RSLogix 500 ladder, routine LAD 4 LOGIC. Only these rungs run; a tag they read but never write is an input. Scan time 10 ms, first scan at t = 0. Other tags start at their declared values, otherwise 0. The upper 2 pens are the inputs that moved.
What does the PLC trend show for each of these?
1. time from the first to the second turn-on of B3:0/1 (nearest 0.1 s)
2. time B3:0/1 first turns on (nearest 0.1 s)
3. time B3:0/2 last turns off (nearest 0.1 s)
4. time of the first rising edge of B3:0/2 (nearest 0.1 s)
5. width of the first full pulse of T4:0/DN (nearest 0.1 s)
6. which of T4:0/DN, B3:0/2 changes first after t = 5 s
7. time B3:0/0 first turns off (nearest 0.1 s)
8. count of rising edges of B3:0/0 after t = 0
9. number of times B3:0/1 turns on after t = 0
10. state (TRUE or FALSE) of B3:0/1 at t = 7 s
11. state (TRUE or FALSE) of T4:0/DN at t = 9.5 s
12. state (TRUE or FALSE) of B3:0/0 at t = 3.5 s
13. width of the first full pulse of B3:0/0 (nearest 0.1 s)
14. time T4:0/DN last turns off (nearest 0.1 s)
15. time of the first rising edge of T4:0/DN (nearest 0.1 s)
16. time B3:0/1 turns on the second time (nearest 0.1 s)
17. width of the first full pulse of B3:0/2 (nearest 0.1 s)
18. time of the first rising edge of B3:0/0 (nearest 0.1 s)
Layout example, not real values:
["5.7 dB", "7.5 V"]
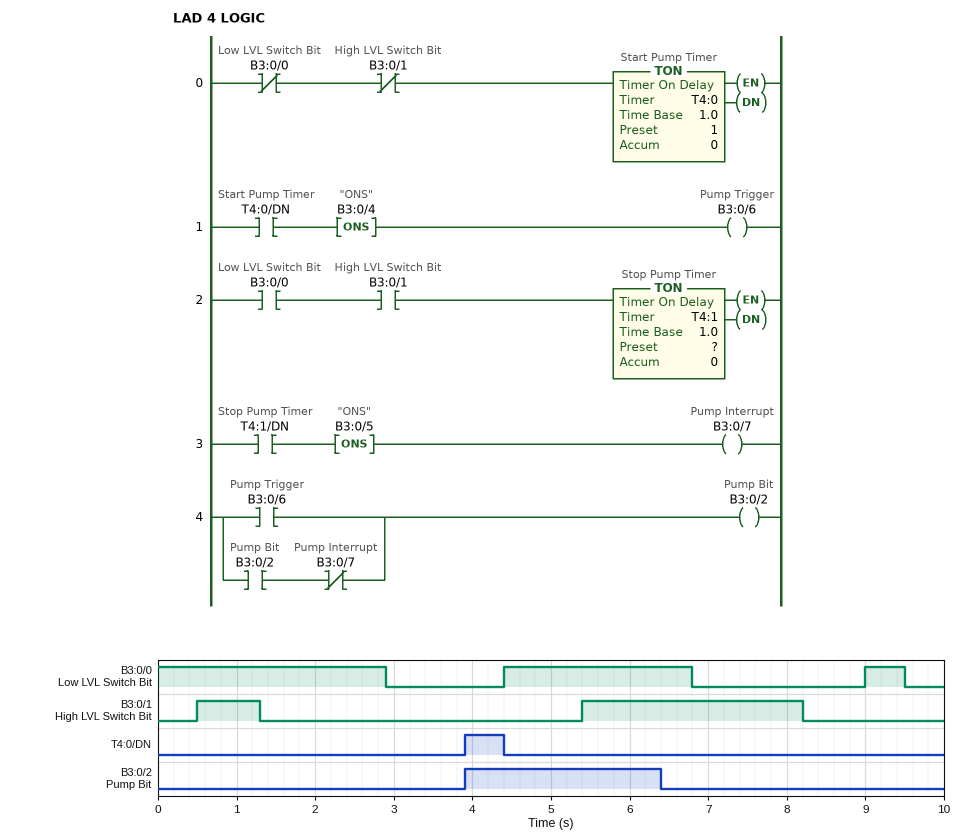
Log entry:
["4.9 s", "0.5 s", "6.4 s", "3.9 s", "0.5 s", "B3:0/2", "2.9 s", "2", "2", "TRUE", "FALSE", "FALSE", "2.4 s", "4.4 s", "3.9 s", "5.4 s", "2.5 s", "4.4 s"]
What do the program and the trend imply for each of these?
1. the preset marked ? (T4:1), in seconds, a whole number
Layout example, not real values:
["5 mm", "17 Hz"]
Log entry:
["1 s"]
